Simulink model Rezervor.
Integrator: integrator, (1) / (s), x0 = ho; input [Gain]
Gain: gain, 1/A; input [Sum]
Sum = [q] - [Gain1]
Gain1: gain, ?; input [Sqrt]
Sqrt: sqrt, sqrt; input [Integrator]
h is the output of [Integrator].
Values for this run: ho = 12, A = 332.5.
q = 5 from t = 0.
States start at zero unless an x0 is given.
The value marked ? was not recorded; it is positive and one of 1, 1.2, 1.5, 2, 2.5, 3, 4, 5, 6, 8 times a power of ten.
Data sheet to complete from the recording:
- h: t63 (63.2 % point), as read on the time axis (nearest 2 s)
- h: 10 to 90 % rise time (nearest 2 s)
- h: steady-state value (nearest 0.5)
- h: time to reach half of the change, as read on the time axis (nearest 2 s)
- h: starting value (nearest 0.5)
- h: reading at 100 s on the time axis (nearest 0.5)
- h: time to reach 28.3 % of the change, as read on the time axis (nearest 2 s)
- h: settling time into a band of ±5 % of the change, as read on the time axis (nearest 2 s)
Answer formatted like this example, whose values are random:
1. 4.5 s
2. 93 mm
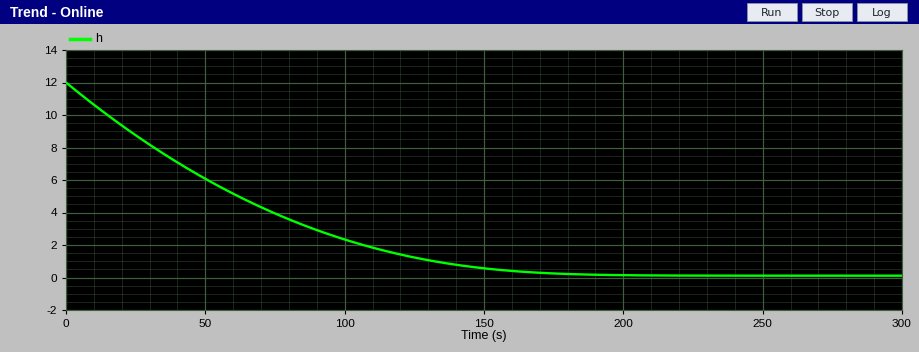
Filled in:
1. 68 s
2. 114 s
3. 0.0
4. 50 s
5. 12.0
6. 2.5
7. 26 s
8. 144 s
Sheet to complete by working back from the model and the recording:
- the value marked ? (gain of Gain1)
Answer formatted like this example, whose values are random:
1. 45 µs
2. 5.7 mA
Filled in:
1. 15
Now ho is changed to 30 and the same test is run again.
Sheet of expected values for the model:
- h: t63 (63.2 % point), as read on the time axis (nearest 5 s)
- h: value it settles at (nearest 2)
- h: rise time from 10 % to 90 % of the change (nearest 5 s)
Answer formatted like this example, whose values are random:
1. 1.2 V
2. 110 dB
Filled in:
1. 105 s
2. 0
3. 170 s
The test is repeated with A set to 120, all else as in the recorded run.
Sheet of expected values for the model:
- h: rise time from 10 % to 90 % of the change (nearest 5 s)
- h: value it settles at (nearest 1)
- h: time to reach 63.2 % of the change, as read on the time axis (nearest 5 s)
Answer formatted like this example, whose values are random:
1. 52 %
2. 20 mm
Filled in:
1. 40 s
2. 0
3. 25 s
